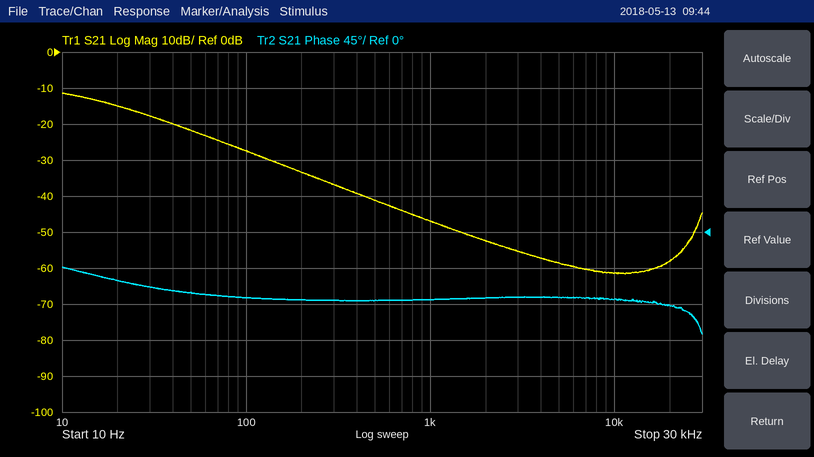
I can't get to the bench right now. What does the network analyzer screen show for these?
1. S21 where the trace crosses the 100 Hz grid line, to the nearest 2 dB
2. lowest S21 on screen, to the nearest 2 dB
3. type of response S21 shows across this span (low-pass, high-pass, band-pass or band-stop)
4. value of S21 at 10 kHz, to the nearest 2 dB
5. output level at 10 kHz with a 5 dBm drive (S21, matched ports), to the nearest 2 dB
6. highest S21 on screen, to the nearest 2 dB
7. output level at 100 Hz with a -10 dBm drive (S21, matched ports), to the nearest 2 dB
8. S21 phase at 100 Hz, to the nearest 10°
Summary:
-28 dB
-62 dB
low-pass
-62 dB
-56 dBm
-12 dB
-38 dBm
-80°
